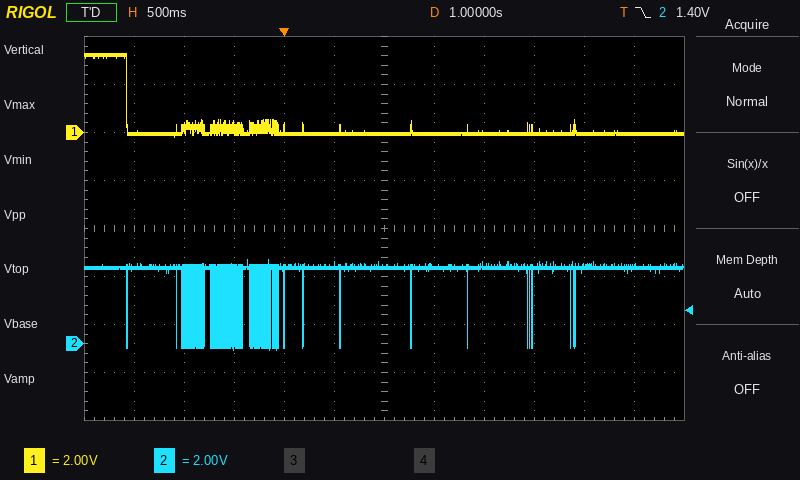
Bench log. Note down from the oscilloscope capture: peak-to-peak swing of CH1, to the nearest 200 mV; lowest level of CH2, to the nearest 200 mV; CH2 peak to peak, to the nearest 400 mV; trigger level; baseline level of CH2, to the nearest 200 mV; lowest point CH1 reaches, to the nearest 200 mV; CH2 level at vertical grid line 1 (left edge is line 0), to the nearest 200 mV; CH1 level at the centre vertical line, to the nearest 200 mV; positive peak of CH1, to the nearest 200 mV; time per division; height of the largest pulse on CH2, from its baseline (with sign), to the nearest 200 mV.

3.4 V
-200 mV
3.6 V
1.40 V
3.2 V
-200 mV
3.2 V
0.0 V
3.2 V
500 ms
-3.4 V
